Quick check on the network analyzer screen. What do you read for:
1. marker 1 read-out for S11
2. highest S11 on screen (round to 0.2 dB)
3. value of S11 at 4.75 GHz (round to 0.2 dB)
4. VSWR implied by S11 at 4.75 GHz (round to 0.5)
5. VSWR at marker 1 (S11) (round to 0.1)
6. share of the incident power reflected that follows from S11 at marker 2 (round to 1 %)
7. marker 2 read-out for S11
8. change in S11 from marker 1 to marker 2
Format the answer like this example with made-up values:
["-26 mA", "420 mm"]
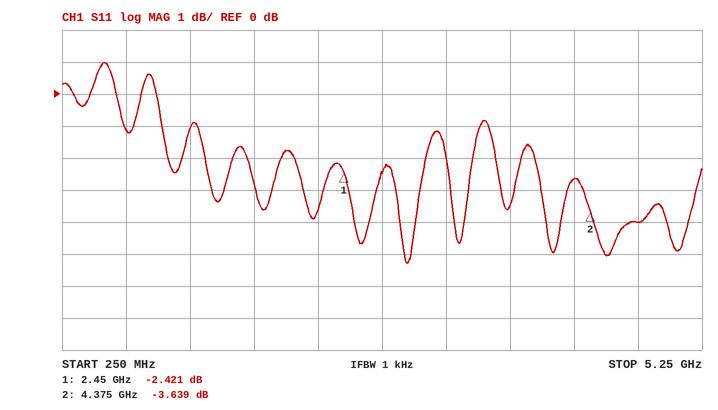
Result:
["-2.421 dB", "1.0 dB", "-4.0 dB", "4.5", "7.2", "43 %", "-3.639 dB", "-1.218 dB"]
